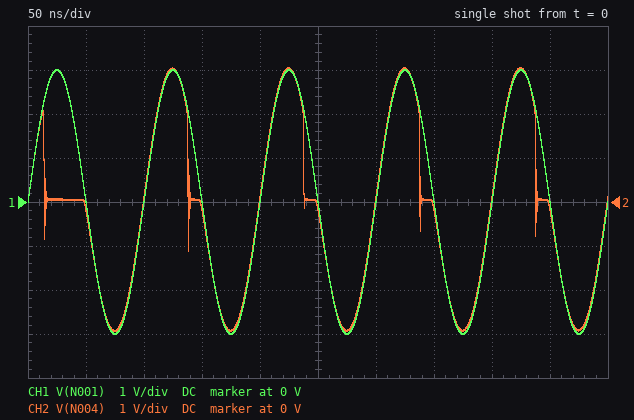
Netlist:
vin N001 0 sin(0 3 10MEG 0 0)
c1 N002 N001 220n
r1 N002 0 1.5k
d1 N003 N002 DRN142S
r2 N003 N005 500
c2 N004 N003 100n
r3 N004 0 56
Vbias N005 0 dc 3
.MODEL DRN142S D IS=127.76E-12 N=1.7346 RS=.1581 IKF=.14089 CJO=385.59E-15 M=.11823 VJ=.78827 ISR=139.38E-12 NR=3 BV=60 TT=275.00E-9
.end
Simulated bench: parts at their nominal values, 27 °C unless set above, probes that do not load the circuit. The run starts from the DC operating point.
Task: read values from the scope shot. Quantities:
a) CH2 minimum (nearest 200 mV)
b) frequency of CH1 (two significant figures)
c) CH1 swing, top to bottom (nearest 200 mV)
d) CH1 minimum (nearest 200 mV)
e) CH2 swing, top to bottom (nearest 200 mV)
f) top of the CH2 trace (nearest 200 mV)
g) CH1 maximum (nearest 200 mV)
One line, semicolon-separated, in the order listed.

-3.0 V; 10 MHz; 6.0 V; -3.0 V; 6.0 V; 3.0 V; 3.0 V
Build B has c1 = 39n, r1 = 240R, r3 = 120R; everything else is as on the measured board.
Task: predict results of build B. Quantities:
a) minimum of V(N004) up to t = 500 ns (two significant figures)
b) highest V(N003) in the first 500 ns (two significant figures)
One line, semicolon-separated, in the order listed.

-3.0 V; 4.5 V
